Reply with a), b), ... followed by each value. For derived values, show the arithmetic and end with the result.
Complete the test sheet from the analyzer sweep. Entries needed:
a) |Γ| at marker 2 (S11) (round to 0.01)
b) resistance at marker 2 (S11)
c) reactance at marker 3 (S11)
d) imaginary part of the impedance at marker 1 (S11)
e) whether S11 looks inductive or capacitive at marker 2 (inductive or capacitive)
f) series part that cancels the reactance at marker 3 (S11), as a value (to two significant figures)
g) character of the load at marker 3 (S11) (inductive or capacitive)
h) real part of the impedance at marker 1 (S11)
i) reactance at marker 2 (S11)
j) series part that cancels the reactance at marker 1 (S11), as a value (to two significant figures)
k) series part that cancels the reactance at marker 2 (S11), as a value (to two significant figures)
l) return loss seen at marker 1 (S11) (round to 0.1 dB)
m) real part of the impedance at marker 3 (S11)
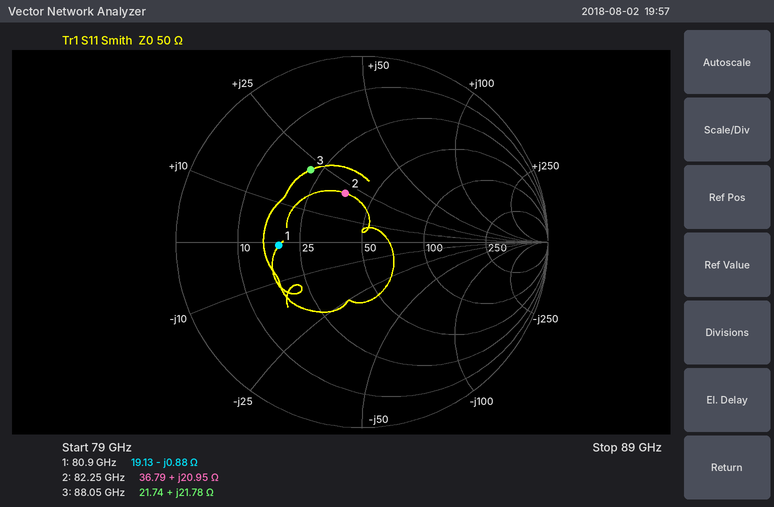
a) 0.28
b) 36.79 Ω
c) +21.78 Ω
d) -0.88 Ω
e) inductive
f) C = 1/(2π × 88.05 GHz × 21.78 Ω) ≈ 83 fF
g) inductive
h) 19.13 Ω
i) +20.95 Ω
j) L = 0.88 Ω/(2π × 80.9 GHz) ≈ 1.7 pH
k) C = 1/(2π × 82.25 GHz × 20.95 Ω) ≈ 92 fF
l) 7.0 dB
m) 21.74 Ω
